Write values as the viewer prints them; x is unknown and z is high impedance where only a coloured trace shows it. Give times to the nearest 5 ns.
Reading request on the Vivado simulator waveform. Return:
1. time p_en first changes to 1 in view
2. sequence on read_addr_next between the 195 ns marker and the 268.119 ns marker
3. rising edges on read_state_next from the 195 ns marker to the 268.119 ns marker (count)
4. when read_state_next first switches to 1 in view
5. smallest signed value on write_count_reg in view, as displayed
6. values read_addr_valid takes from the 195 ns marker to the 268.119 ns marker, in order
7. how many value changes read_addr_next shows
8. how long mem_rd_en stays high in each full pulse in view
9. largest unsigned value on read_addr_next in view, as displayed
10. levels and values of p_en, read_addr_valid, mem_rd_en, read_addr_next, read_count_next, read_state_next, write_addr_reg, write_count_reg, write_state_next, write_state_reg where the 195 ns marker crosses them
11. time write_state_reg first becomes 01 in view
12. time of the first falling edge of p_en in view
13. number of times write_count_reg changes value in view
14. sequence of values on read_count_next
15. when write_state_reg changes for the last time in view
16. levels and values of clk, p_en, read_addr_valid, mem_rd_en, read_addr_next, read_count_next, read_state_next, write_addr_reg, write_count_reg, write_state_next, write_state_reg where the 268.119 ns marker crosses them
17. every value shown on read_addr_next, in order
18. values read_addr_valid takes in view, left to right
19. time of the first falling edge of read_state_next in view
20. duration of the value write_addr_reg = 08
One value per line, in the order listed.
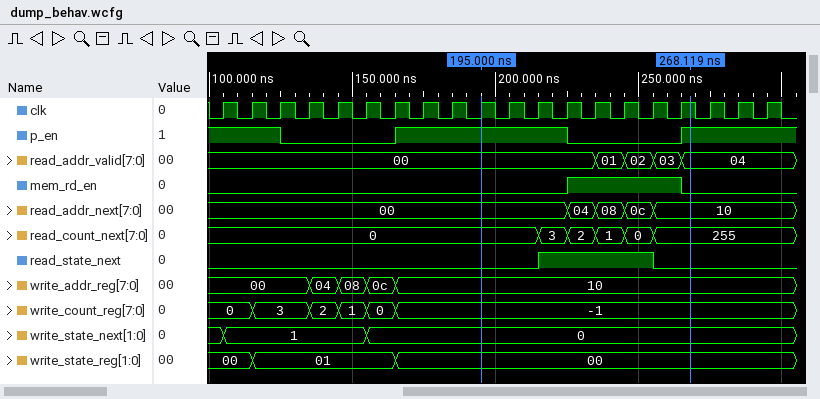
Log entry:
165 ns
00, 04, 08, 0c, 10
1
215 ns
-1
00, 01, 02, 03, 04
4
40 ns
10
p_en=1, read_addr_valid=00, mem_rd_en=0, read_addr_next=00, read_count_next=0, read_state_next=0, write_addr_reg=10, write_count_reg=-1, write_state_next=0, write_state_reg=00
115 ns
125 ns
5
0, 3, 2, 1, 0, 255
165 ns
clk=1, p_en=1, read_addr_valid=04, mem_rd_en=0, read_addr_next=10, read_count_next=255, read_state_next=0, write_addr_reg=10, write_count_reg=-1, write_state_next=0, write_state_reg=00
00, 04, 08, 0c, 10
00, 01, 02, 03, 04
255 ns
10 ns
